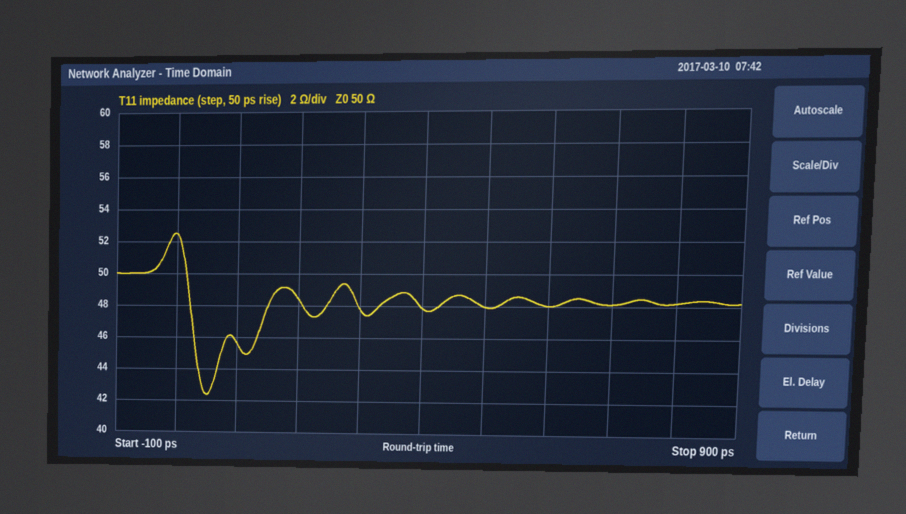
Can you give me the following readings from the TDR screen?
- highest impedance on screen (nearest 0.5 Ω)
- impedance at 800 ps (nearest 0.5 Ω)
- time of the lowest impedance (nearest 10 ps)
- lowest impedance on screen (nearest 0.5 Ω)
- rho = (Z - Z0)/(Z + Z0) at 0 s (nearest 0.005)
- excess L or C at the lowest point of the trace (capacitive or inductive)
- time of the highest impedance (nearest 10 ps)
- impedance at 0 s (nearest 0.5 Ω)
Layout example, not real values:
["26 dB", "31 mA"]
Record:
["52.5 Ω", "48.0 Ω", "50 ps", "42.5 Ω", "+0.025", "capacitive", "0 ps", "52.5 Ω"]
